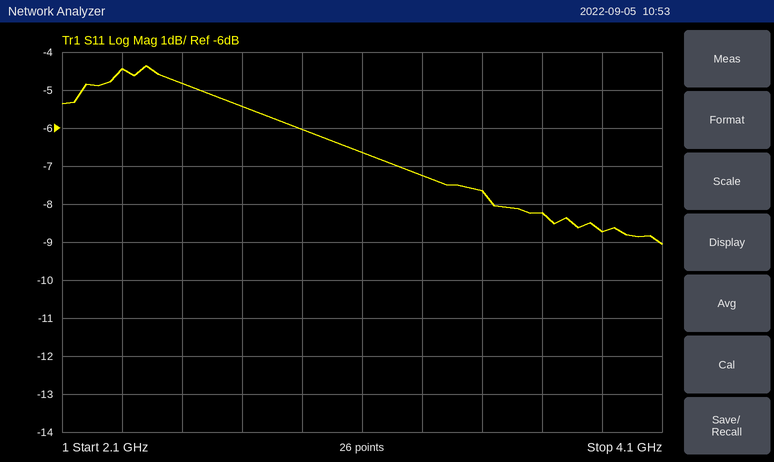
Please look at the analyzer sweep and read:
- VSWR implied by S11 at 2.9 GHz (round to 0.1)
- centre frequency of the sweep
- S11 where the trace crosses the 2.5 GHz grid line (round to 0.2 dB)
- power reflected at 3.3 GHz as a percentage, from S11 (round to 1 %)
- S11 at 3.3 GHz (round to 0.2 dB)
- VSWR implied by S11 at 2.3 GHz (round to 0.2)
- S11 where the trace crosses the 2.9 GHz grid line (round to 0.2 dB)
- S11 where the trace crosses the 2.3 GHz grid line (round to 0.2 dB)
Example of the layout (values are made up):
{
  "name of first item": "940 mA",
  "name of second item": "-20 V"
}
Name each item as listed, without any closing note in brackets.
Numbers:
{
  "VSWR implied by S11 at 2.9 GHz": "3.0",
  "centre frequency of the sweep": "3.1 GHz",
  "S11 where the trace crosses the 2.5 GHz grid line": "-4.8 dB",
  "power reflected at 3.3 GHz as a percentage, from S11": "19 %",
  "S11 at 3.3 GHz": "-7.2 dB",
  "VSWR implied by S11 at 2.3 GHz": "4.0",
  "S11 where the trace crosses the 2.9 GHz grid line": "-6.0 dB",
  "S11 where the trace crosses the 2.3 GHz grid line": "-4.4 dB"
}
